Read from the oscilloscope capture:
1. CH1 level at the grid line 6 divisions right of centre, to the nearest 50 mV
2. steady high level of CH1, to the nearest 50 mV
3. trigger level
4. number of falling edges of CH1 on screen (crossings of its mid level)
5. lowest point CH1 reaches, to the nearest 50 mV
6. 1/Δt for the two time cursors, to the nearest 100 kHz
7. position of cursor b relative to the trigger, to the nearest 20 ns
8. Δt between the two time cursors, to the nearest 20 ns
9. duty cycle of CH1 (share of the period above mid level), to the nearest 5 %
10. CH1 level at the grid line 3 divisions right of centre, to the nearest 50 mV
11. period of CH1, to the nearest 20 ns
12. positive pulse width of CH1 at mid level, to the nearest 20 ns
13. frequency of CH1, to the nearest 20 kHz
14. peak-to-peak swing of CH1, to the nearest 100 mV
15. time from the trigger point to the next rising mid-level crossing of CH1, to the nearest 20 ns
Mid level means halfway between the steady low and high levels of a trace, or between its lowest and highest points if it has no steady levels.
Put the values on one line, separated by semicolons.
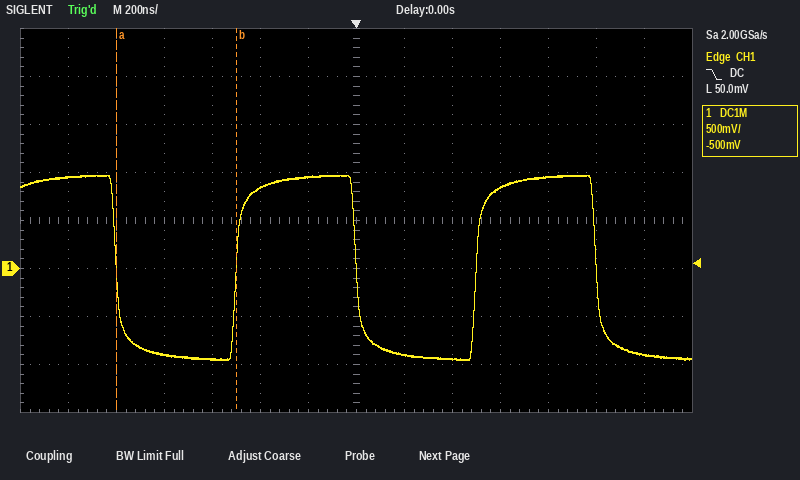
-900 mV; 950 mV; 50.0 mV; 3; -950 mV; 2.0 MHz; -500 ns; 500 ns; 50 %; 850 mV; 1.00 µs; 500 ns; 1.00 MHz; 1.90 V; 500 ns
